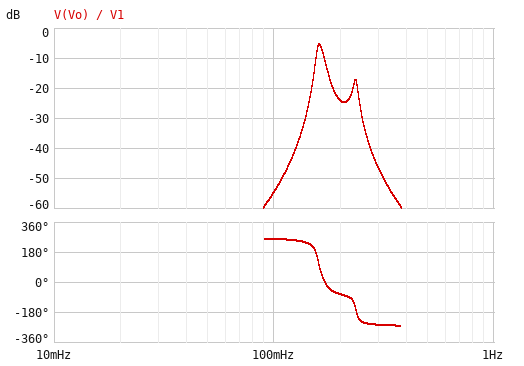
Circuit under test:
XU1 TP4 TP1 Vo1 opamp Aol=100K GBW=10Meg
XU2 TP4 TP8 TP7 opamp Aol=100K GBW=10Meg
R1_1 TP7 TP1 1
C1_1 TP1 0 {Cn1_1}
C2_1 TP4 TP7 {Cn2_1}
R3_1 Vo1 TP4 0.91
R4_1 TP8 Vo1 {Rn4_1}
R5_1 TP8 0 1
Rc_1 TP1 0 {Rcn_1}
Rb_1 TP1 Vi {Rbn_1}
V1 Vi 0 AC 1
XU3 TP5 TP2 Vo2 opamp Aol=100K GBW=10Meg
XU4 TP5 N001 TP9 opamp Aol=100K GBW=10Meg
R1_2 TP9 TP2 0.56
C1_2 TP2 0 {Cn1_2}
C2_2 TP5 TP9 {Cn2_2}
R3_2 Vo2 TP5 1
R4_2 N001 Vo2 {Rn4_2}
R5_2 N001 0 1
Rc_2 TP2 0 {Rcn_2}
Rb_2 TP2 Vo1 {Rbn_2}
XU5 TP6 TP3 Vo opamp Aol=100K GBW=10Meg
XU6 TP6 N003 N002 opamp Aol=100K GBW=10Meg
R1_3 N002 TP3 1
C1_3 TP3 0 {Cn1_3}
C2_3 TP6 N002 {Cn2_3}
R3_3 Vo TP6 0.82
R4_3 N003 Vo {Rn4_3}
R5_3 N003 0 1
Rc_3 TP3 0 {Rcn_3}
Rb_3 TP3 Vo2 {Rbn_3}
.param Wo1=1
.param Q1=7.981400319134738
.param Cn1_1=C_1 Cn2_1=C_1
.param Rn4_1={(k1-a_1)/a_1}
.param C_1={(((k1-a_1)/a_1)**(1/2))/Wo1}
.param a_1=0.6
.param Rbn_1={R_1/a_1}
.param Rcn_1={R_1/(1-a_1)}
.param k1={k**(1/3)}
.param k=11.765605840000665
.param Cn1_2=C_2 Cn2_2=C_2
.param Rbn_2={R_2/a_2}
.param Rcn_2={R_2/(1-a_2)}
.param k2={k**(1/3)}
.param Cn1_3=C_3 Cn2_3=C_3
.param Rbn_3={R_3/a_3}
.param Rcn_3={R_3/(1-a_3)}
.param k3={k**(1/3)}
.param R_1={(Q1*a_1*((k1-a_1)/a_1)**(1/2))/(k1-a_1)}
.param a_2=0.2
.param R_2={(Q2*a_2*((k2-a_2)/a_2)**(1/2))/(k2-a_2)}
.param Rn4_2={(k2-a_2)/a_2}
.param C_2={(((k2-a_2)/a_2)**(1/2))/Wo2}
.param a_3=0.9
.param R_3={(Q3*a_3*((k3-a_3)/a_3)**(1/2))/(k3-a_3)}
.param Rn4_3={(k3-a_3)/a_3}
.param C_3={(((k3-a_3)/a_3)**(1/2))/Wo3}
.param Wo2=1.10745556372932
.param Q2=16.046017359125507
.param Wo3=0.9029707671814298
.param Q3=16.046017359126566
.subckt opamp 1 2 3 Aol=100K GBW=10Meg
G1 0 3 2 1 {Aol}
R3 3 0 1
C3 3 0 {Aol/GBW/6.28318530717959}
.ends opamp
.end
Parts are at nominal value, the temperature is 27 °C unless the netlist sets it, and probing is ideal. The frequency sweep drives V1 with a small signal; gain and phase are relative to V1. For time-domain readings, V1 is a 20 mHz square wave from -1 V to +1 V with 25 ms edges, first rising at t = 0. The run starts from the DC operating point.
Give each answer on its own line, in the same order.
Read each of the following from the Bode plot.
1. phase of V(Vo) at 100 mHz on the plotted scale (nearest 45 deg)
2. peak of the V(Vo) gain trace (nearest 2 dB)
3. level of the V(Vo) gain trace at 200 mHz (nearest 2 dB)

270 deg
-6 dB
-24 dB
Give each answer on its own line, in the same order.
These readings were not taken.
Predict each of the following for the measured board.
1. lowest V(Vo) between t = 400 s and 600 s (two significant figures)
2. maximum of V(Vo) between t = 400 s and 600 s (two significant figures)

-27 mV
27 mV
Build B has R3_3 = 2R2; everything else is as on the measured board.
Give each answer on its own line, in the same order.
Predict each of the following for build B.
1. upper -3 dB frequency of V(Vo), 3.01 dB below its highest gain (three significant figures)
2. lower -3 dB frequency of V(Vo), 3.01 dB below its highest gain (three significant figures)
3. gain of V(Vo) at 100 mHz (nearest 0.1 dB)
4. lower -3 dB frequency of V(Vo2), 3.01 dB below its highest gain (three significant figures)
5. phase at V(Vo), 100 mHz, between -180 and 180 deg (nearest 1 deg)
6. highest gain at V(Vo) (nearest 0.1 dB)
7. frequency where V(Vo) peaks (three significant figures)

240 mHz
229 mHz
-31.7 dB
229 mHz
138 deg
-20.9 dB
235 mHz
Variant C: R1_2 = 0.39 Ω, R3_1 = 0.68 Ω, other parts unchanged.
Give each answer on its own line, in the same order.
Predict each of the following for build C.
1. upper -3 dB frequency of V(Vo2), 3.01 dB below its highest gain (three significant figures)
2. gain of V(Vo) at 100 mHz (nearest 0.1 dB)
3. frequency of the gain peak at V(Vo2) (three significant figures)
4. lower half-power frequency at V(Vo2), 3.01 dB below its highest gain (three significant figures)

287 mHz
-62.0 dB
282 mHz
276 mHz
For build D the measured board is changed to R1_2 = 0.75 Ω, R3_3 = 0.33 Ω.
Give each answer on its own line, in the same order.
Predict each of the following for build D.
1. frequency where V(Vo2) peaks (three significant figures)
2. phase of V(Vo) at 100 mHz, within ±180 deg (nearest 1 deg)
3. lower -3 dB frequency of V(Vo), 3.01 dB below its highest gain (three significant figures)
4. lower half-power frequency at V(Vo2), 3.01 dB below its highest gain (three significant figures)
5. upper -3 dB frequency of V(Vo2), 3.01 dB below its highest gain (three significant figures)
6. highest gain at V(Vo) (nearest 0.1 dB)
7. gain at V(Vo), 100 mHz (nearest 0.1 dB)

203 mHz
-99 deg
198 mHz
196 mHz
208 mHz
-10.8 dB
-62.2 dB
